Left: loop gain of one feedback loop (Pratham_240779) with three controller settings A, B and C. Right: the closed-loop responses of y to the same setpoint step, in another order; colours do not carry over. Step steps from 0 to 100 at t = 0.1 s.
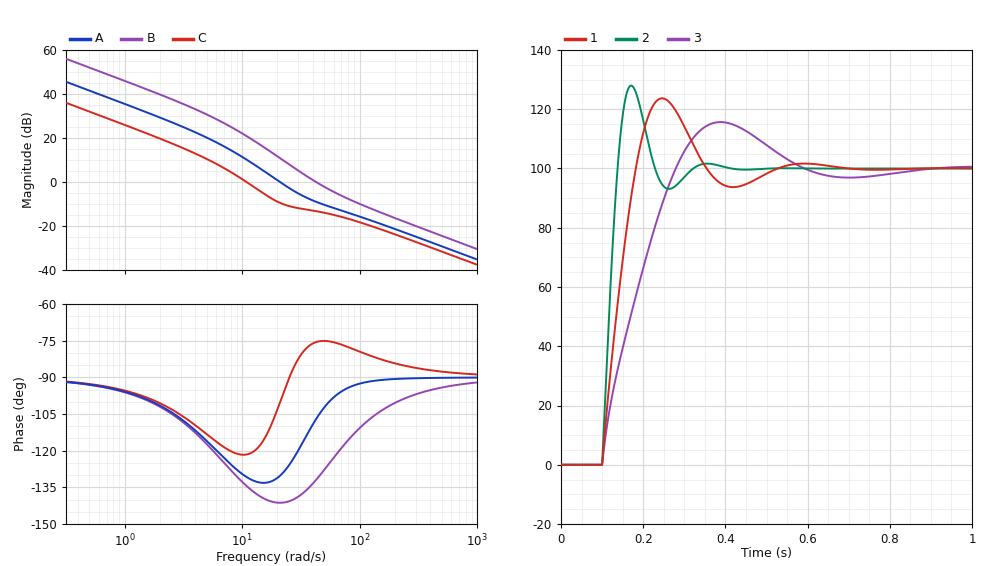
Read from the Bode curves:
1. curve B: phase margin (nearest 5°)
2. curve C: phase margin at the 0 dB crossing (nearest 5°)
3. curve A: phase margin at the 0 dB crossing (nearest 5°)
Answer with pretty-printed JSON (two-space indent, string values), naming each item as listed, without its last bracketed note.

{
  "curve B: phase margin": "50°",
  "curve C: phase margin at the 0 dB crossing": "60°",
  "curve A: phase margin at the 0 dB crossing": "50°"
}
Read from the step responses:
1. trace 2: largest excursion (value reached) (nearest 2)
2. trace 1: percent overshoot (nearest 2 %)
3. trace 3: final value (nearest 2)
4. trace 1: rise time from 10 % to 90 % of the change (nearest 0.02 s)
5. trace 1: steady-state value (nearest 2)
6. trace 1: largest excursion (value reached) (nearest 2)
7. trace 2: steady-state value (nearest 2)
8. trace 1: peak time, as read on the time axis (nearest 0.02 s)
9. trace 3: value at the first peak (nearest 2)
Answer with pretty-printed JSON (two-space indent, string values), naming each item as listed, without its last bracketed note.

{
  "trace 2: largest excursion (value reached)": "128",
  "trace 1: percent overshoot": "24 %",
  "trace 3: final value": "100",
  "trace 1: rise time from 10 % to 90 % of the change": "0.06 s",
  "trace 1: steady-state value": "100",
  "trace 1: largest excursion (value reached)": "124",
  "trace 2: steady-state value": "100",
  "trace 1: peak time, as read on the time axis": "0.24 s",
  "trace 3: value at the first peak": "116"
}
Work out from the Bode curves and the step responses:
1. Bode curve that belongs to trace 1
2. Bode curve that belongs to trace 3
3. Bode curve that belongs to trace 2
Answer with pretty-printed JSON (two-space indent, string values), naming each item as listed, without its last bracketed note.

{
  "Bode curve that belongs to trace 1": "A",
  "Bode curve that belongs to trace 3": "C",
  "Bode curve that belongs to trace 2": "B"
}
